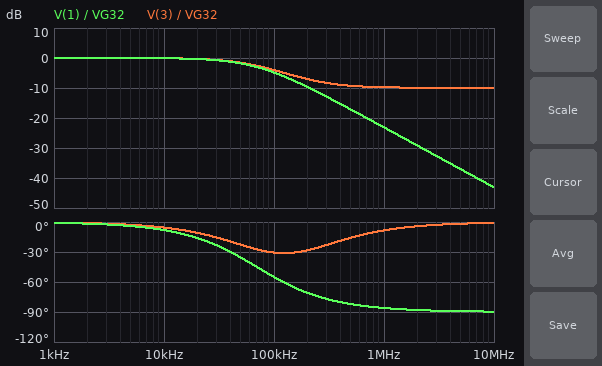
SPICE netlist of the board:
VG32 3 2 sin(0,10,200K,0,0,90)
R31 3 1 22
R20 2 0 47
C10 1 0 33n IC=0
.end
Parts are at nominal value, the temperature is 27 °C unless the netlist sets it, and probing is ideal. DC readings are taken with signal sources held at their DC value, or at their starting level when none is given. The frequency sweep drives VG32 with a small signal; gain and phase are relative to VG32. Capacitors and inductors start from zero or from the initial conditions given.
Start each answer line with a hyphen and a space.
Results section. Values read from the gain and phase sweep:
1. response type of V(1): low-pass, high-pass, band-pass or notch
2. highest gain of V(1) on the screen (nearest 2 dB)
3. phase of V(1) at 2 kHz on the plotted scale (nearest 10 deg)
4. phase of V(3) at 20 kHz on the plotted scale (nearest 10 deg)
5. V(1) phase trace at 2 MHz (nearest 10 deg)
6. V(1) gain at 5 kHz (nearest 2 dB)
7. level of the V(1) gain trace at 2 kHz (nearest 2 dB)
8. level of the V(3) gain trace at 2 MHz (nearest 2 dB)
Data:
- low-pass
- 0 dB
- 0 deg
- -10 deg
- -90 deg
- 0 dB
- 0 dB
- -10 dB
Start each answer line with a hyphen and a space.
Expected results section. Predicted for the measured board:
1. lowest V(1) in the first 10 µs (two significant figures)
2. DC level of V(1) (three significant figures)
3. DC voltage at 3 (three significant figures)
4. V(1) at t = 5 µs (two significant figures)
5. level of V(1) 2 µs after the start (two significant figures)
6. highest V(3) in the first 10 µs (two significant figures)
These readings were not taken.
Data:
- -3.5 V
- 10.0 V
- 10.0 V
- 970 mV
- 500 mV
- 4.4 V
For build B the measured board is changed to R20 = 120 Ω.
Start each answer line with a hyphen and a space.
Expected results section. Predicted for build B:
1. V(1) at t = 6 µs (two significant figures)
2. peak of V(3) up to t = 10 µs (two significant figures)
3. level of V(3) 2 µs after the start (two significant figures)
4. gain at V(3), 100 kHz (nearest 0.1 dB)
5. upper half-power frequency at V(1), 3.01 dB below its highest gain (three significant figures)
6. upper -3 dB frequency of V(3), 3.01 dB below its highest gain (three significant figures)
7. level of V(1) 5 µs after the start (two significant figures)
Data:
- 1.6 V
- 2.2 V
- -780 mV
- -9.0 dB
- 34.0 kHz
- 34.8 kHz
- 180 mV
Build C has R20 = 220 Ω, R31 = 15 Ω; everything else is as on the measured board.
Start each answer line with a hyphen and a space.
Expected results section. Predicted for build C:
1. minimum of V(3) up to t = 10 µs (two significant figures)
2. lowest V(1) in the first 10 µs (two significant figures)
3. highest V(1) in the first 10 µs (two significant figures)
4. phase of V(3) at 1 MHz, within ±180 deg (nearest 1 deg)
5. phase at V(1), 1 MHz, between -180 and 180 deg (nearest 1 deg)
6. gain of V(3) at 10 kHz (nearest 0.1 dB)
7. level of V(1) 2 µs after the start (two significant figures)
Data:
- -1.3 V
- -1.1 V
- 970 mV
- -17 deg
- -89 deg
- -0.9 dB
- 430 mV
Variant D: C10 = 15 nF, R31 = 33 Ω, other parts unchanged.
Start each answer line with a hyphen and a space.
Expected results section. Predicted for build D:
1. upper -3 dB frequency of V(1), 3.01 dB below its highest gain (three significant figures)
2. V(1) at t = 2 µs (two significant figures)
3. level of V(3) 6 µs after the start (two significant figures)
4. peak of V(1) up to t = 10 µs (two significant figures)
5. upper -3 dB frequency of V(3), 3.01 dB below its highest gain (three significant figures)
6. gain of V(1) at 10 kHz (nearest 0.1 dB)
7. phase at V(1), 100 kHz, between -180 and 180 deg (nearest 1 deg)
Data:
- 133 kHz
- -340 mV
- 4.4 V
- 5.5 V
- 163 kHz
- 0 dB
- -37 deg
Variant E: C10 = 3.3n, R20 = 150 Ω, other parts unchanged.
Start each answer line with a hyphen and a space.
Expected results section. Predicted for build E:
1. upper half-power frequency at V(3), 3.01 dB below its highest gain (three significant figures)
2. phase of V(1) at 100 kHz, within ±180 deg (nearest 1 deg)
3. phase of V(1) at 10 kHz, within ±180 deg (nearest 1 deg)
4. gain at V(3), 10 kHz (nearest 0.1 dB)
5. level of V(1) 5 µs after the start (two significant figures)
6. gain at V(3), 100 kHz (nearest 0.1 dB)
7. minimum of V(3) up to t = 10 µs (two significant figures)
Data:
- 285 kHz
- -20 deg
- -2 deg
- 0 dB
- 6.6 V
- -0.5 dB
- -8.2 V
